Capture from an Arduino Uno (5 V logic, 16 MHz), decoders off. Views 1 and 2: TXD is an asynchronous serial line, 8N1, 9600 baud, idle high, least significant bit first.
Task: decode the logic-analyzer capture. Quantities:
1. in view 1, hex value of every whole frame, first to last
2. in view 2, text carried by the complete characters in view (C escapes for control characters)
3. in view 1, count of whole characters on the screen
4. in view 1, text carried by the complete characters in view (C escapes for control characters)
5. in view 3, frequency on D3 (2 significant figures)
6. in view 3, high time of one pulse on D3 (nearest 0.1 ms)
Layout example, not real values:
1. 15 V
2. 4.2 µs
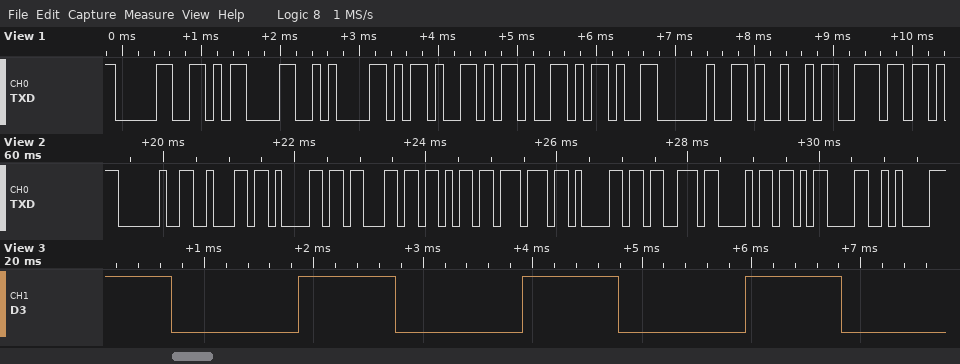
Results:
1. 30 0D 0A 2D 2D 2D 20 49 6E
2. " backwash\r\n"
3. 9
4. "0\r\n--- In"
5. 490 Hz
6. 0.9 ms
